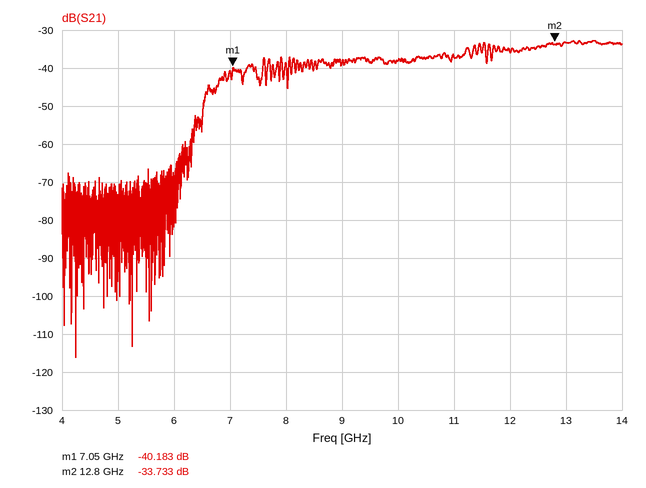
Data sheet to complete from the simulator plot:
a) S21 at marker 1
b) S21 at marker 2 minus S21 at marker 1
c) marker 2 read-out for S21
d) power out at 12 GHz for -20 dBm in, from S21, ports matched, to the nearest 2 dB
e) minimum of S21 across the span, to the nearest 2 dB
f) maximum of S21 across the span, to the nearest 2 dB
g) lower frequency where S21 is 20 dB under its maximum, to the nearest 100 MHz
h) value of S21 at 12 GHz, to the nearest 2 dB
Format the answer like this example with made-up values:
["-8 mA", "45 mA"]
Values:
["-40.183 dB", "6.450 dB", "-33.733 dB", "-56 dBm", "-116 dB", "-32 dB", "6.5 GHz", "-36 dB"]
